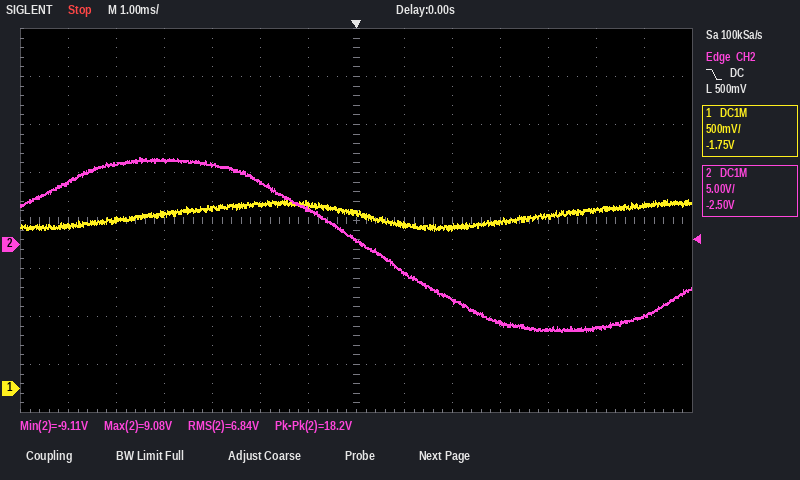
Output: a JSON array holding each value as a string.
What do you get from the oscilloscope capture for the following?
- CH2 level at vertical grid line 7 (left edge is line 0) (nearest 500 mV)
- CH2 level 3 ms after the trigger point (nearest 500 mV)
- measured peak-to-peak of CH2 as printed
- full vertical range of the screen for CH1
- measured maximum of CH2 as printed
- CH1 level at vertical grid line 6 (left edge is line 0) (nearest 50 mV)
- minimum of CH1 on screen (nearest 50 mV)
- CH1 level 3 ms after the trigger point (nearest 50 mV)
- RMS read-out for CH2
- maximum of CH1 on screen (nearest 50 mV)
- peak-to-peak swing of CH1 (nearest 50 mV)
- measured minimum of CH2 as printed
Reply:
["500 mV", "-8.0 V", "18.2 V", "4 V", "9.08 V", "1.90 V", "1.65 V", "1.75 V", "6.84 V", "1.95 V", "300 mV", "-9.11 V"]
